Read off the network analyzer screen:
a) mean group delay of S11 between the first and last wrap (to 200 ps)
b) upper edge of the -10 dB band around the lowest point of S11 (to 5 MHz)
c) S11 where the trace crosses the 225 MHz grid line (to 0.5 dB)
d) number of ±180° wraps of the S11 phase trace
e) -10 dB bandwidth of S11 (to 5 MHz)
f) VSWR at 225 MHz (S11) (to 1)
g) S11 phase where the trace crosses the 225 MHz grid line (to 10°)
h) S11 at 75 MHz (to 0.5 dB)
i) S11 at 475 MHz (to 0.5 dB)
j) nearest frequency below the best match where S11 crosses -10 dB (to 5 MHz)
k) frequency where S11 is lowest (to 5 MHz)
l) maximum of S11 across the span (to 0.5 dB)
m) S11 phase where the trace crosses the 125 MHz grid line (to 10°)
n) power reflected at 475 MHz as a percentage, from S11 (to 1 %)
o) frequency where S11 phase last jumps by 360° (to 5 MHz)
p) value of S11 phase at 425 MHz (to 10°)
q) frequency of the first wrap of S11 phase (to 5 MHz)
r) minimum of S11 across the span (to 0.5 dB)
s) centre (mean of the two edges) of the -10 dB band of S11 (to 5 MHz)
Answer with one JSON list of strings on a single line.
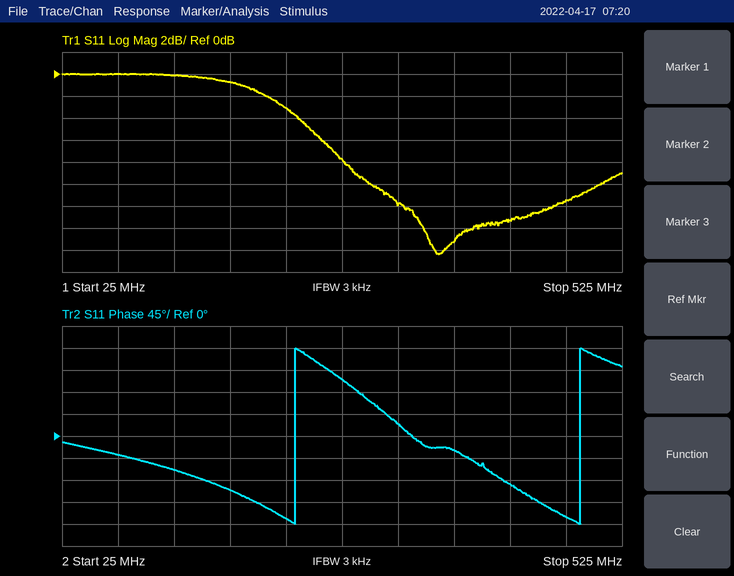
["4.0 ns", "505 MHz", "-3.0 dB", "2", "205 MHz", "6", "-170°", "0.0 dB", "-11.5 dB", "300 MHz", "360 MHz", "0.0 dB", "-70°", "7 %", "490 MHz", "-100°", "235 MHz", "-16.5 dB", "405 MHz"]
